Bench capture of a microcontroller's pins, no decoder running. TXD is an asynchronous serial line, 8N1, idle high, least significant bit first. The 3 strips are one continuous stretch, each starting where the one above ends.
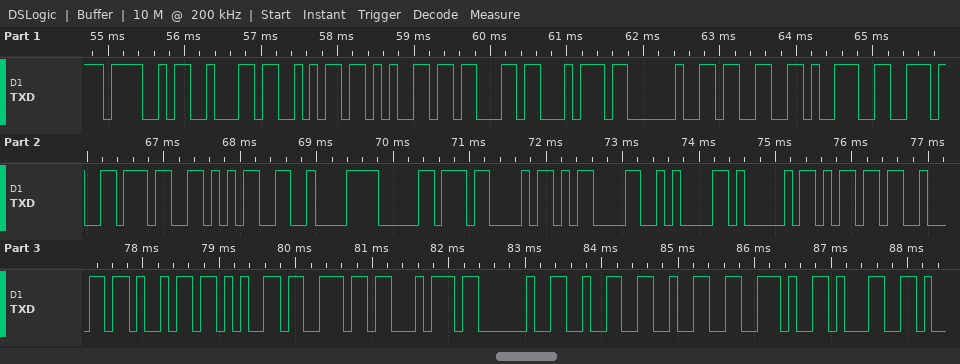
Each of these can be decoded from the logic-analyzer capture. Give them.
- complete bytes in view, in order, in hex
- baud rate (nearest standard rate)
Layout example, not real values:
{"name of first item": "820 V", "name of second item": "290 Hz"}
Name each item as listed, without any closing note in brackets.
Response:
{"complete bytes in view, in order, in hex": "4F 62 6A 65 63 74 20 33 39 2E 37 35 C2 B0 43 0D 0A 41 6D 62 69 65 6E 74 20 32 32 2E 31", "baud rate": "9600 baud"}
